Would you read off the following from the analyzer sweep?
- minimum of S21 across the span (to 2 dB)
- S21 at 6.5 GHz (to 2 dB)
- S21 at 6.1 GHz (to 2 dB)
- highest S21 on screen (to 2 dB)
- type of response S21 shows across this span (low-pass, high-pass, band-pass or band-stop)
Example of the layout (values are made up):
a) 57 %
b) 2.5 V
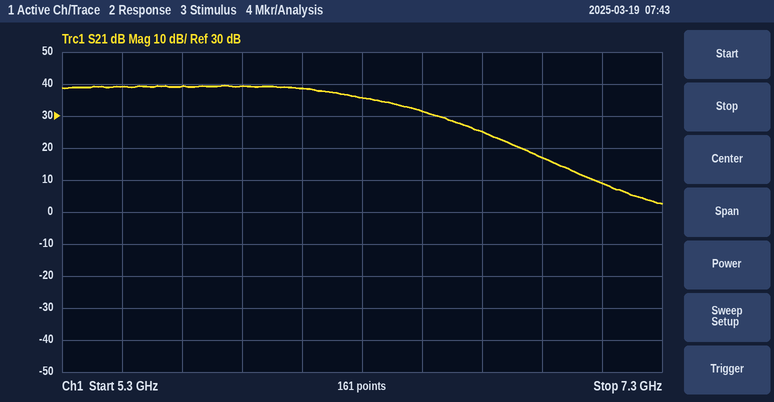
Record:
a) 2 dB
b) 32 dB
c) 38 dB
d) 40 dB
e) low-pass
